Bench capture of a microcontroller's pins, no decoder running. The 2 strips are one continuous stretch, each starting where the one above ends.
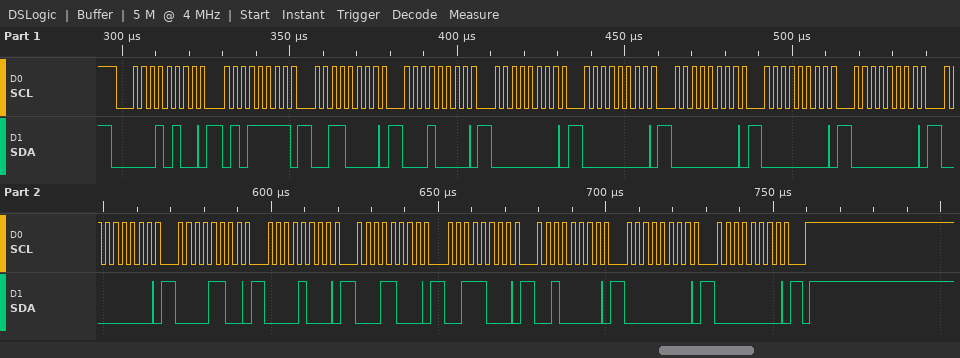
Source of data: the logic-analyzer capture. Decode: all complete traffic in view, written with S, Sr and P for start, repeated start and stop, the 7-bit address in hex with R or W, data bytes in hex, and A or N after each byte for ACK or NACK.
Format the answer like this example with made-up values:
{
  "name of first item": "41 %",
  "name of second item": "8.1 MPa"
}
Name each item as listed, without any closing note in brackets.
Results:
{
  "all complete traffic in view, written with S, Sr and P for start, repeated start and stop, the 7-bit address in hex with R or W, data bytes in hex, and A or N after each byte for ACK or NACK": "S 0AW A 5F A 30 A 10 A 00 A 00 A 00 A 00 A 00 A 00 A 0C A 08 A 18 A 38 A 20 A 00 A 00 A P"
}
